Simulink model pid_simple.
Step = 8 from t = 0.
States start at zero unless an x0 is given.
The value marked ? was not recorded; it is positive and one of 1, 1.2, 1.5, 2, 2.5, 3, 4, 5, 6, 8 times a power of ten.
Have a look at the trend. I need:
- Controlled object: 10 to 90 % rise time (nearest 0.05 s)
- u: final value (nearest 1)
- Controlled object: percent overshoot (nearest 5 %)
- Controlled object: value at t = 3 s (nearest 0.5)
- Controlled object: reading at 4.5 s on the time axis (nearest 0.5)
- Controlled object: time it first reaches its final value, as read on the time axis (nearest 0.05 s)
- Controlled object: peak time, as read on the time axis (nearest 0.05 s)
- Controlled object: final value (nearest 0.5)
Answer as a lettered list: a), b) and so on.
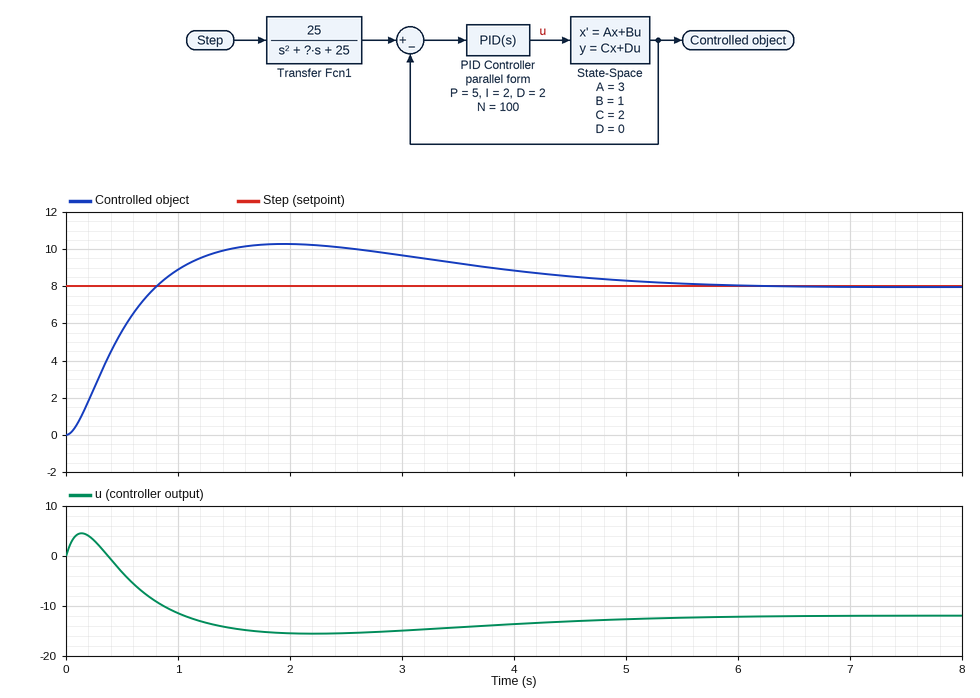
a) 0.55 s
b) -12
c) 30 %
d) 9.5
e) 8.5
f) 0.80 s
g) 1.95 s
h) 8.0
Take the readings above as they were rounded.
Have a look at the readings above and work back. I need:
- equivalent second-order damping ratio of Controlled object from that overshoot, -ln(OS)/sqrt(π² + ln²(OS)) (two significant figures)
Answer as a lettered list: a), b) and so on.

a) 0.36
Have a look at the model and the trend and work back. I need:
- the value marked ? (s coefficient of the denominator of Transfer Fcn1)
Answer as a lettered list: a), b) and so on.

a) 10
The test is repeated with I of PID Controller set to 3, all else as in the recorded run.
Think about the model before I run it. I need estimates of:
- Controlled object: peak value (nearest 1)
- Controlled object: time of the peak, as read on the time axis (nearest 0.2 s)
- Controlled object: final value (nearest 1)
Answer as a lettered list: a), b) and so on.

a) 10
b) 1.8 s
c) 8
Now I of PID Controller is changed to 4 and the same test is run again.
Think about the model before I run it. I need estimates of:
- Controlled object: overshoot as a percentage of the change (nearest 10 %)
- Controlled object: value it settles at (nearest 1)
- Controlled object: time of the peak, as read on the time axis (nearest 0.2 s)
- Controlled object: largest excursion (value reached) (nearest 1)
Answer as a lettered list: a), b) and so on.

a) 20 %
b) 8
c) 1.6 s
d) 10
